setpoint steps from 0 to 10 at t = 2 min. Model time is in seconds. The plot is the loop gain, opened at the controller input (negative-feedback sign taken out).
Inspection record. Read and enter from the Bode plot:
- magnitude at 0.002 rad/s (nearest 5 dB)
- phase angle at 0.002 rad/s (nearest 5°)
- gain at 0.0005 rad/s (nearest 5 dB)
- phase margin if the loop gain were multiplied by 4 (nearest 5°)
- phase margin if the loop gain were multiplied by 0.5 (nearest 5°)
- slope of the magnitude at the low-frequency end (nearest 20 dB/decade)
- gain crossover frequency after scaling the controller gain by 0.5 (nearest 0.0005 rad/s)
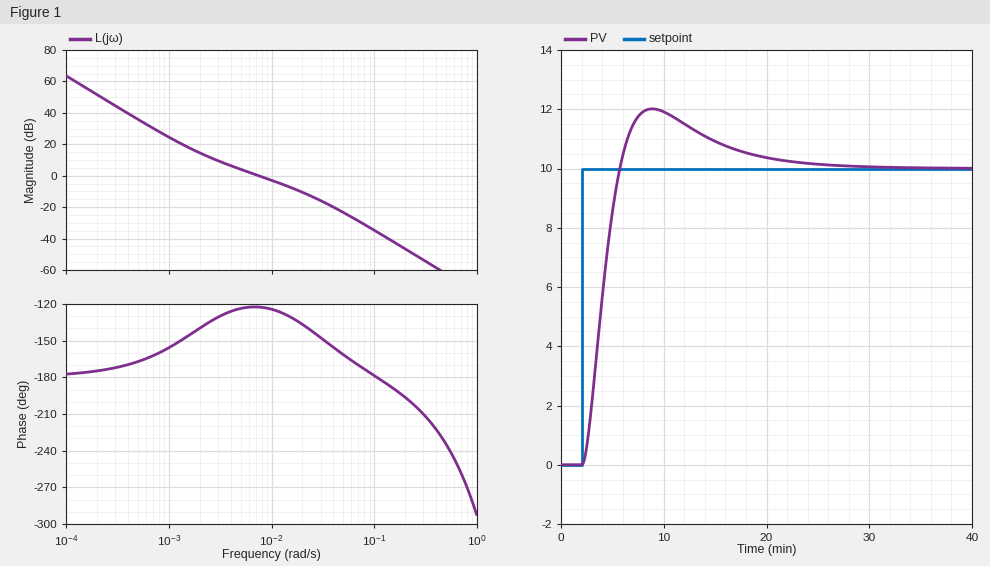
15 dB
-140°
35 dB
40°
55°
-40 dB/decade
0.0040 rad/s
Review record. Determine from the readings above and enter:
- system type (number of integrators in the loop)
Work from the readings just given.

2
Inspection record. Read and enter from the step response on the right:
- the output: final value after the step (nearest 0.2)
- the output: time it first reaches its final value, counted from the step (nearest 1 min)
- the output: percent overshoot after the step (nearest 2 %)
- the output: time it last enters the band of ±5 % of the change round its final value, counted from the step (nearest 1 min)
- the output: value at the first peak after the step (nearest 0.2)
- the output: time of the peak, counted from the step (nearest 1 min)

10.0
4 min
20 %
16 min
12.0
7 min
